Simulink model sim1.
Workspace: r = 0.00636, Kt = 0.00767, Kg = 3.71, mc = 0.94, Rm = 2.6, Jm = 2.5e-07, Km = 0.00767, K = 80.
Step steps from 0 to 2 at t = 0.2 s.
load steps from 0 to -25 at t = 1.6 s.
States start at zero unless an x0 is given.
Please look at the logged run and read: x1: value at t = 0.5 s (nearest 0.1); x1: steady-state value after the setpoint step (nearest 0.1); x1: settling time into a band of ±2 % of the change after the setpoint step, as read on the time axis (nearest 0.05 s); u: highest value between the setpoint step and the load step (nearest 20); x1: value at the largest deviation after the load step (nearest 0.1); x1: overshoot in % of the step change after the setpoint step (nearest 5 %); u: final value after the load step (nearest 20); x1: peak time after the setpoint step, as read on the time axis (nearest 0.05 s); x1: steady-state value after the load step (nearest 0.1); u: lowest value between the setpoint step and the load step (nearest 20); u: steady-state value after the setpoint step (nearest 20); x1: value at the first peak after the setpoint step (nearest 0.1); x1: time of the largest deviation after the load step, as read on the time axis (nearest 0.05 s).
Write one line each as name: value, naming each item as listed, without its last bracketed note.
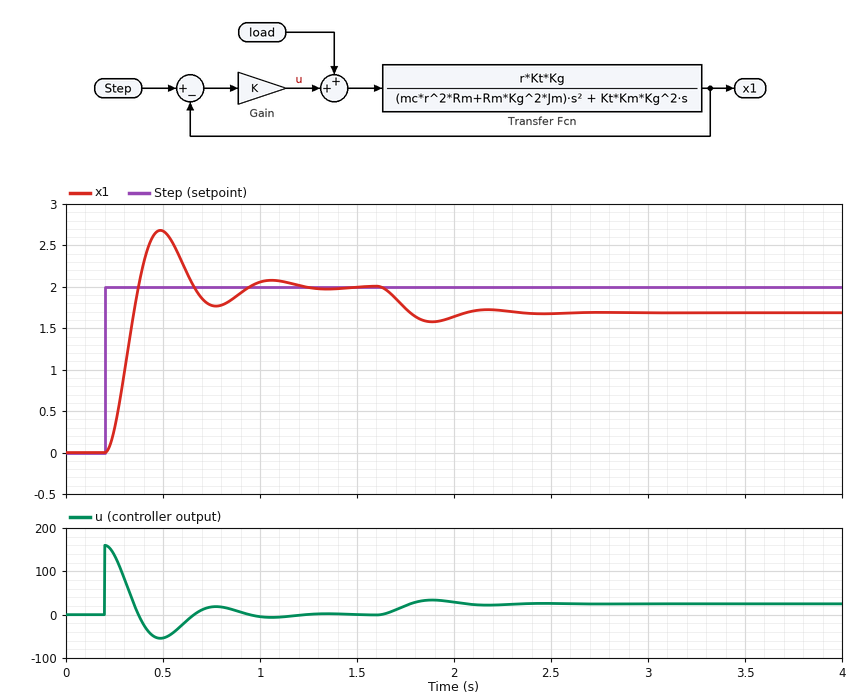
x1: value at t = 0.5 s: 2.7
x1: steady-state value after the setpoint step: 2.0
x1: settling time into a band of ±2 % of the change after the setpoint step, as read on the time axis: 1.15 s
u: highest value between the setpoint step and the load step: 160
x1: value at the largest deviation after the load step: 1.6
x1: overshoot in % of the step change after the setpoint step: 35 %
u: final value after the load step: 20
x1: peak time after the setpoint step, as read on the time axis: 0.50 s
x1: steady-state value after the load step: 1.7
u: lowest value between the setpoint step and the load step: -60
u: steady-state value after the setpoint step: 0
x1: value at the first peak after the setpoint step: 2.7
x1: time of the largest deviation after the load step, as read on the time axis: 1.90 s
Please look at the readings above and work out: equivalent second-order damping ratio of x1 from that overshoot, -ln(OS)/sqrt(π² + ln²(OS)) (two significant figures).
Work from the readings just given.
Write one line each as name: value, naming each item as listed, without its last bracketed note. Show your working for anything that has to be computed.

equivalent second-order damping ratio of x1 from that overshoot, -ln(OS)/sqrt(π² + ln²(OS)): ln(0.35) = -1.050; 1.050 / sqrt(9.870 + 1.102) = 0.32
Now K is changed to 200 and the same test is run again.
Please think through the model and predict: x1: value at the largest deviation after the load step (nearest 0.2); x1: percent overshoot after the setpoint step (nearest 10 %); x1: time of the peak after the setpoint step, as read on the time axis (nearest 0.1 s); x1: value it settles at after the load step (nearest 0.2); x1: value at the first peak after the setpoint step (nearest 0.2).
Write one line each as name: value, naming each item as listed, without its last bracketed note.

x1: value at the largest deviation after the load step: 1.8
x1: percent overshoot after the setpoint step: 50 %
x1: time of the peak after the setpoint step, as read on the time axis: 0.4 s
x1: value it settles at after the load step: 1.8
x1: value at the first peak after the setpoint step: 3.0
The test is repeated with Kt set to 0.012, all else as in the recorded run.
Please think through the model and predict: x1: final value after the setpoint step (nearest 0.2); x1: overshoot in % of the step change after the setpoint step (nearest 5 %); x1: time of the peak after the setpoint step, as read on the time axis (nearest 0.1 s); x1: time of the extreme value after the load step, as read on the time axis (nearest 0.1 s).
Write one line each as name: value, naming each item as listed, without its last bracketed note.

x1: final value after the setpoint step: 2.0
x1: overshoot in % of the step change after the setpoint step: 25 %
x1: time of the peak after the setpoint step, as read on the time axis: 0.4 s
x1: time of the extreme value after the load step, as read on the time axis: 1.8 s
